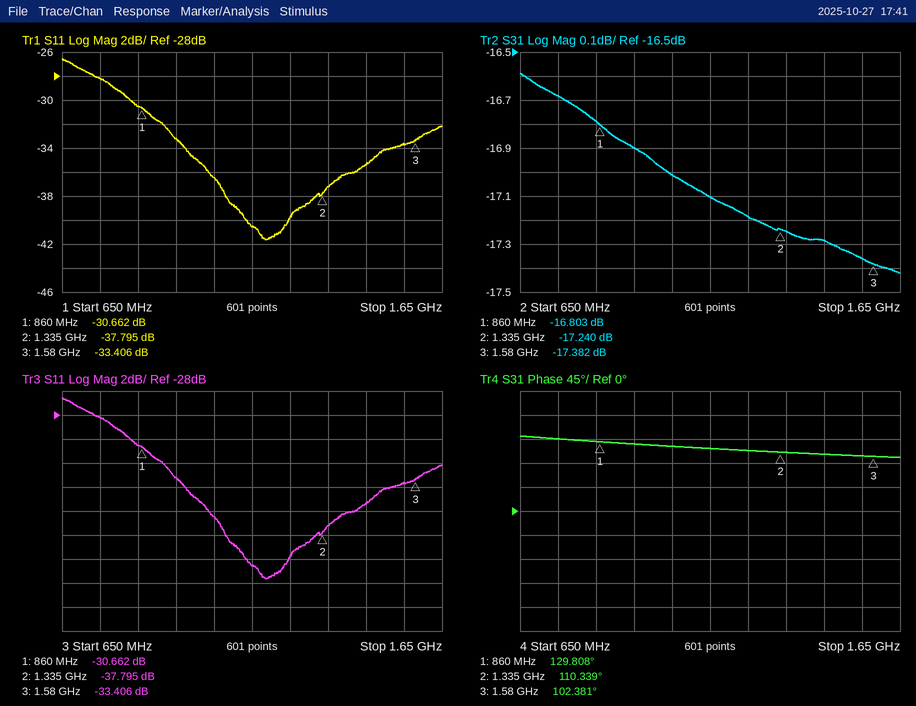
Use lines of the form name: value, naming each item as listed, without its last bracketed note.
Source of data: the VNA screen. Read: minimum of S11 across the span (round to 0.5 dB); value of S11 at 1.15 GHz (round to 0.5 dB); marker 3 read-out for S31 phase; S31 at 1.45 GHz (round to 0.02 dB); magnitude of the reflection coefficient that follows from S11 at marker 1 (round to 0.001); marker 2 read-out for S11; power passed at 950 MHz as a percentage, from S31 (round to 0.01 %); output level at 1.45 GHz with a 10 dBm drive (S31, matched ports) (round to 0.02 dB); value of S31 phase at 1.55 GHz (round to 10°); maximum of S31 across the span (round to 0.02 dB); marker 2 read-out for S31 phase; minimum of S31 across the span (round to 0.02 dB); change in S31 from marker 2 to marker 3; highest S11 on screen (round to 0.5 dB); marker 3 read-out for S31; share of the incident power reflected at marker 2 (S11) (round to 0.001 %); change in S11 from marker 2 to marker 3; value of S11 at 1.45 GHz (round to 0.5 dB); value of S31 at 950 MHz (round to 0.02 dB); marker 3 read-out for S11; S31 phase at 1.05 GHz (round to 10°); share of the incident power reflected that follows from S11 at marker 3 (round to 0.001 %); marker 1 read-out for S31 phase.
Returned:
minimum of S11 across the span: -41.5 dB
value of S11 at 1.15 GHz: -40.5 dB
marker 3 read-out for S31 phase: 102.381°
S31 at 1.45 GHz: -17.28 dB
magnitude of the reflection coefficient that follows from S11 at marker 1: 0.029
marker 2 read-out for S11: -37.795 dB
power passed at 950 MHz as a percentage, from S31: 2.04 %
output level at 1.45 GHz with a 10 dBm drive (S31, matched ports): -7.28 dBm
value of S31 phase at 1.55 GHz: 100°
maximum of S31 across the span: -16.58 dB
marker 2 read-out for S31 phase: 110.339°
minimum of S31 across the span: -17.42 dB
change in S31 from marker 2 to marker 3: -0.142 dB
highest S11 on screen: -26.5 dB
marker 3 read-out for S31: -17.382 dB
share of the incident power reflected at marker 2 (S11): 0.017 %
change in S11 from marker 2 to marker 3: 4.389 dB
value of S11 at 1.45 GHz: -35.5 dB
value of S31 at 950 MHz: -16.90 dB
marker 3 read-out for S11: -33.406 dB
S31 phase at 1.05 GHz: 120°
share of the incident power reflected that follows from S11 at marker 3: 0.046 %
marker 1 read-out for S31 phase: 129.808°
